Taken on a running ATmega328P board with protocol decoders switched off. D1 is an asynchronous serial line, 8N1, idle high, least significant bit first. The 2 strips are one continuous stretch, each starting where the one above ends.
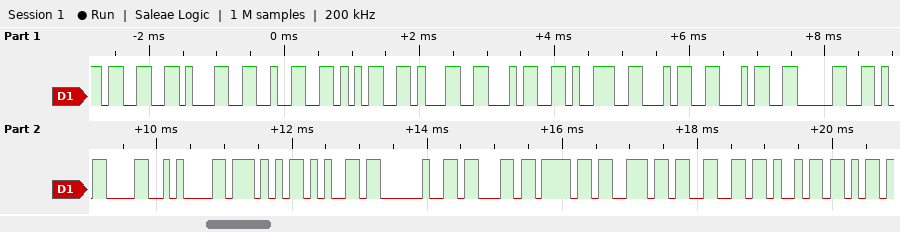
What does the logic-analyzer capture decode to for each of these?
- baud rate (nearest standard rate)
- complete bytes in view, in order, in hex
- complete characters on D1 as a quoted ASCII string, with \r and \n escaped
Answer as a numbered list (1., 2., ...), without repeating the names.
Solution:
1. 9600 baud
2. 33 31 32 35 31 34 39 34 34 30 0D 0A 57 65 20 63 6F 6E 66 69
3. "3125149440\r\nWe confi"
